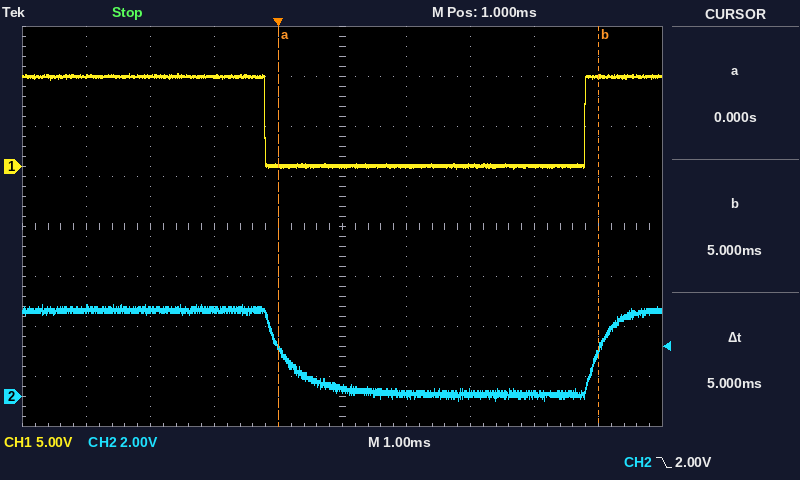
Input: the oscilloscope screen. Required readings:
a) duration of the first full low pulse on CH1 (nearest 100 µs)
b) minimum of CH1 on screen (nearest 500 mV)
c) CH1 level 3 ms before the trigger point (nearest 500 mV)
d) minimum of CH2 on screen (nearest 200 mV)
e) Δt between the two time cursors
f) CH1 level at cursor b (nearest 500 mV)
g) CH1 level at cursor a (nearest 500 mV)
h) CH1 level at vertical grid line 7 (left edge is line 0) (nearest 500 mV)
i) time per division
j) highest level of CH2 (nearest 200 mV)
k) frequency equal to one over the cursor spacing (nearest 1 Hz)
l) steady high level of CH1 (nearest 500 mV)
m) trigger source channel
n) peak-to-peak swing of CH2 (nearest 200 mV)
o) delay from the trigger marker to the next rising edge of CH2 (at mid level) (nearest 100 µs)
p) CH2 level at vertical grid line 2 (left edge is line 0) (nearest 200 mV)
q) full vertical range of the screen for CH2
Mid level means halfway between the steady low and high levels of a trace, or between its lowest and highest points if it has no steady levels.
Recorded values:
5.0 ms
0.0 V
9.0 V
-200 mV
5 ms
9.0 V
0.0 V
0.0 V
1 ms
3.6 V
200 Hz
9.0 V
CH2
3.8 V
5.0 ms
3.4 V
16 V
